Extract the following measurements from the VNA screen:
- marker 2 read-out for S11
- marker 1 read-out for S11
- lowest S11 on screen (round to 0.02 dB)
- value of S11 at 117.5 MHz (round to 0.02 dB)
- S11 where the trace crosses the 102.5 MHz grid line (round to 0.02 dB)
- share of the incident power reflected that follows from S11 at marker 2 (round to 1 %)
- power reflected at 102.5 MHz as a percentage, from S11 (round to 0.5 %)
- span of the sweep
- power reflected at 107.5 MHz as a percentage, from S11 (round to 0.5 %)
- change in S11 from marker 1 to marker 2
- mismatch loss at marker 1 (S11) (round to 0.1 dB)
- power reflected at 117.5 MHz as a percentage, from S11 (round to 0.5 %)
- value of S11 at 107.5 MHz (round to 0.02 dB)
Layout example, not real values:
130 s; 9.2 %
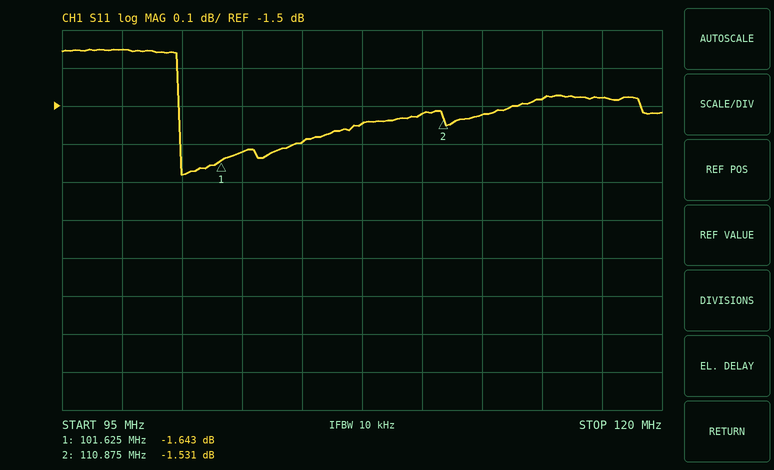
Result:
-1.531 dB; -1.643 dB; -1.68 dB; -1.48 dB; -1.62 dB; 70 %; 69.0 %; 25 MHz; 70.0 %; 0.112 dB; 5.0 dB; 71.0 %; -1.54 dB
